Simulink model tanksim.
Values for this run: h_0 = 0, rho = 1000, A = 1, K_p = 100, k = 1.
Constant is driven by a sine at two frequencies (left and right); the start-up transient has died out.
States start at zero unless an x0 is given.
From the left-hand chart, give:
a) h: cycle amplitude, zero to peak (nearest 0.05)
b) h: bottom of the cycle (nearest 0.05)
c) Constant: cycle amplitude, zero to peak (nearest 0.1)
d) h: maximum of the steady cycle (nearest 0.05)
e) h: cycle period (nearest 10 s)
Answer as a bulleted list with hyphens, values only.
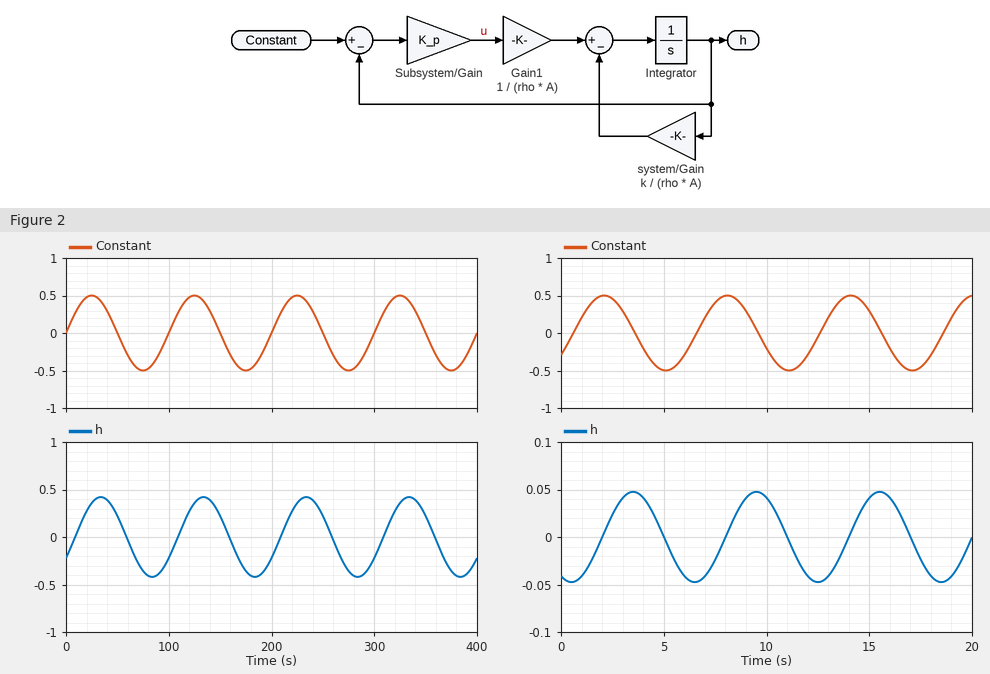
- 0.40
- -0.40
- 0.5
- 0.40
- 100 s
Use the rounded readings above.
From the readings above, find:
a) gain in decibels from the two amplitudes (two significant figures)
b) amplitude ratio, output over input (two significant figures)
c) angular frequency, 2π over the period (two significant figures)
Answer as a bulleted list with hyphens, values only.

- -1.9 dB
- 0.80
- 0.063 rad/s
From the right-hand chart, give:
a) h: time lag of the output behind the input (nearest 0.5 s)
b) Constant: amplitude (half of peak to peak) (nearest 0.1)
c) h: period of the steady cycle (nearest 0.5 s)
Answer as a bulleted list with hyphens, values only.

- 1.5 s
- 0.5
- 6.0 s
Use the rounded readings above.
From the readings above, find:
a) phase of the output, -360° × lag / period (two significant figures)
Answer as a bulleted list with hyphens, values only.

- -90°
